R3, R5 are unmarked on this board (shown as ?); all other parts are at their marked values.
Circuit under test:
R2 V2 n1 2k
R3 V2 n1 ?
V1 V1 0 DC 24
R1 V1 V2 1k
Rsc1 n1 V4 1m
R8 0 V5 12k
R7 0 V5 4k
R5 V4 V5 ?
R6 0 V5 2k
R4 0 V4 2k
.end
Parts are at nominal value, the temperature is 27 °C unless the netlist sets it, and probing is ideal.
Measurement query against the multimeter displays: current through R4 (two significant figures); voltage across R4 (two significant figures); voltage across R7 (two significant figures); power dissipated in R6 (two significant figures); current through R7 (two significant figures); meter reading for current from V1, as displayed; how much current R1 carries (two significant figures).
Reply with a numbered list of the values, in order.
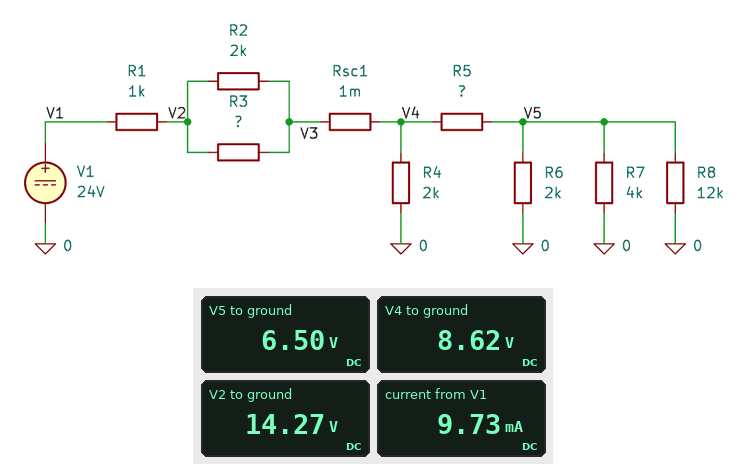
1. 4.3 mA
2. 8.6 V
3. 6.5 V
4. 21 mW
5. 1.6 mA
6. 9.73 mA
7. 9.7 mA
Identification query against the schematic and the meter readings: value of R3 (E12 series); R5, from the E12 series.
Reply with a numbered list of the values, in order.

1. 820 Ω
2. 390 Ω
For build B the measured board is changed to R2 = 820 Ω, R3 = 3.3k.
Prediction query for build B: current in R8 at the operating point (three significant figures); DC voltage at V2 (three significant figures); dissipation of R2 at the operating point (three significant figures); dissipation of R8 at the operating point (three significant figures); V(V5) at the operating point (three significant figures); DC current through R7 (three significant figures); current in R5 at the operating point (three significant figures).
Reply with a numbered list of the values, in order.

1. 526 µA
2. 14.6 V
3. 46.9 mW
4. 3.32 mW
5. 6.31 V
6. 1.58 mA
7. 5.26 mA
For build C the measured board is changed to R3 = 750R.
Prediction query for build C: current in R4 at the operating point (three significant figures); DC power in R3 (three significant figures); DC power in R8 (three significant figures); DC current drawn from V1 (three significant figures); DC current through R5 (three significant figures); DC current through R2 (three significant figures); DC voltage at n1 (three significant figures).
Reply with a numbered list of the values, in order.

1. 4.37 mA
2. 38.7 mW
3. 3.63 mW
4. 9.87 mA
5. 5.50 mA
6. 2.69 mA
7. 8.74 V
